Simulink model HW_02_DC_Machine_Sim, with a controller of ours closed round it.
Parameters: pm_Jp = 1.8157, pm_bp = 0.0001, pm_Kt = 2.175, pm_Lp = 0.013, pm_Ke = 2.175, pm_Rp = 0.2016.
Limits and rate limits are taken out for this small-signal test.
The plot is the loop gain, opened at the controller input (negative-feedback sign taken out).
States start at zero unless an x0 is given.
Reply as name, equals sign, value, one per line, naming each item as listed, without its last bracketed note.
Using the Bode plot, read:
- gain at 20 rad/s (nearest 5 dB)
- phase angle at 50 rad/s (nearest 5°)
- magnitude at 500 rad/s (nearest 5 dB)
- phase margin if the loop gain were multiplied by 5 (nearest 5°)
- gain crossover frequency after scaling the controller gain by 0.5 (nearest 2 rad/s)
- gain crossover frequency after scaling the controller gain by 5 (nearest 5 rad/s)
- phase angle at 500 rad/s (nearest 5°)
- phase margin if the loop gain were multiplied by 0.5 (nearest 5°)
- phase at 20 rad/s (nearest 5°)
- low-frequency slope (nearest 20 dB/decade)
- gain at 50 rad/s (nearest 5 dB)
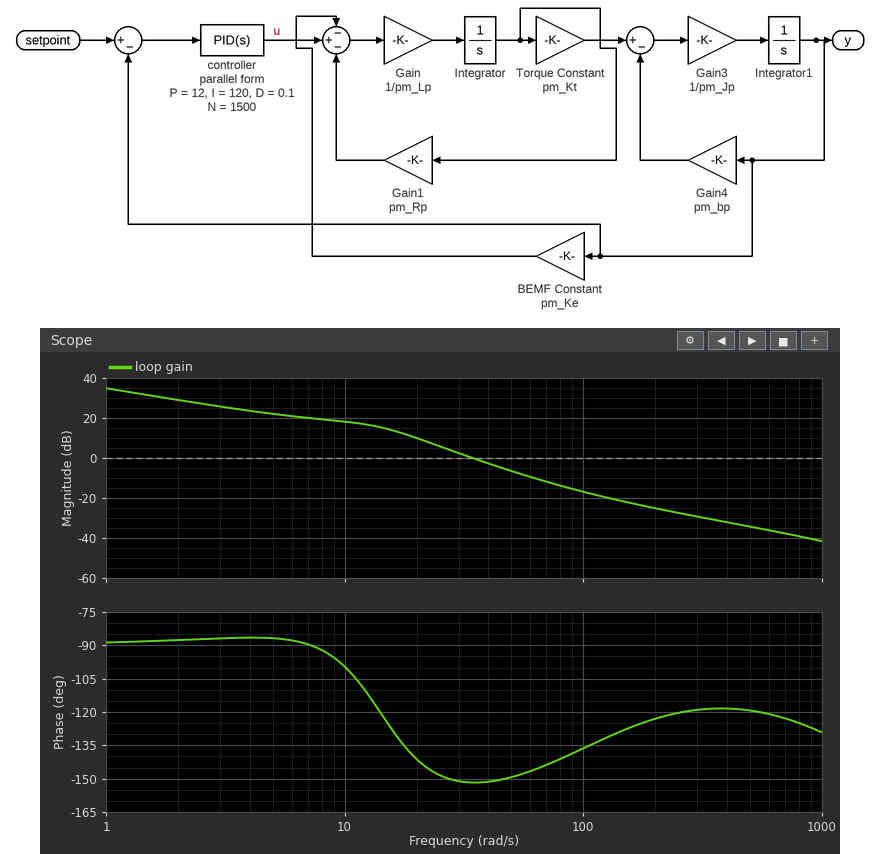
gain at 20 rad/s = 10 dB
phase angle at 50 rad/s = -150°
magnitude at 500 rad/s = -35 dB
phase margin if the loop gain were multiplied by 5 = 40°
gain crossover frequency after scaling the controller gain by 0.5 = 24 rad/s
gain crossover frequency after scaling the controller gain by 5 = 80 rad/s
phase angle at 500 rad/s = -120°
phase margin if the loop gain were multiplied by 0.5 = 30°
phase at 20 rad/s = -140°
low-frequency slope = -20 dB/decade
gain at 50 rad/s = -5 dB
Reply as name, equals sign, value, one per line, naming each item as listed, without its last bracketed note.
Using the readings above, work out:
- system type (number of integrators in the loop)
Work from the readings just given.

system type = 1
